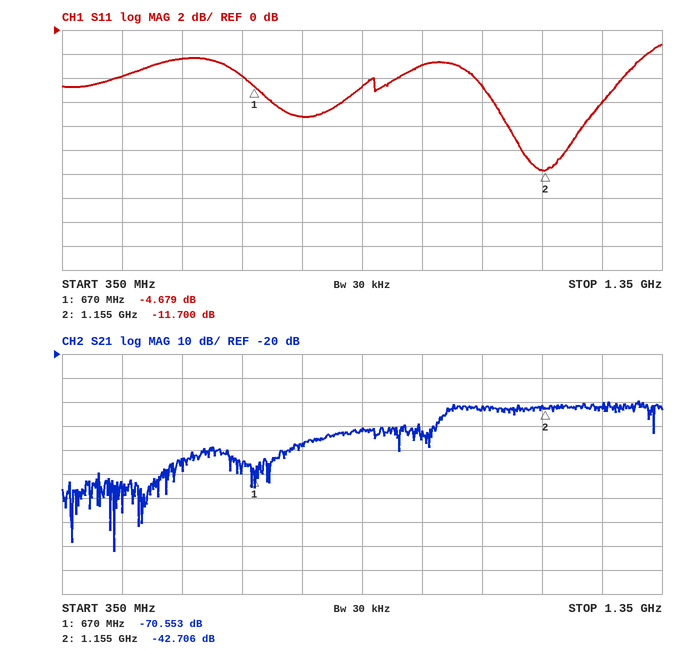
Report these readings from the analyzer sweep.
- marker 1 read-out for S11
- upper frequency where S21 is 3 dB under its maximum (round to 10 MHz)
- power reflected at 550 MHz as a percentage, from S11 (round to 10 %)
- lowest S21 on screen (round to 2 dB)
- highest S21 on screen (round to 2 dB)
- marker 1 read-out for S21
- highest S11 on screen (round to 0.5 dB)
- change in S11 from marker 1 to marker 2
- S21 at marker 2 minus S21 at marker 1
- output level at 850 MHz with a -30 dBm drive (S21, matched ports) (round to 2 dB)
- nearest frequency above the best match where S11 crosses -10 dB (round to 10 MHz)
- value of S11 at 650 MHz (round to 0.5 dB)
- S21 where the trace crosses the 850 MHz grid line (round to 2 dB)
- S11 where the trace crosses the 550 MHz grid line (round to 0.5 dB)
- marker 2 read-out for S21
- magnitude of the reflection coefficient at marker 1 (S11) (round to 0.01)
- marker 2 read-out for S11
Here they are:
-4.679 dB
1.33 GHz
60 %
-102 dB
-40 dB
-70.553 dB
-1.0 dB
-7.021 dB
27.847 dB
-82 dBm
1.19 GHz
-4.0 dB
-52 dB
-2.5 dB
-42.706 dB
0.58
-11.700 dB
